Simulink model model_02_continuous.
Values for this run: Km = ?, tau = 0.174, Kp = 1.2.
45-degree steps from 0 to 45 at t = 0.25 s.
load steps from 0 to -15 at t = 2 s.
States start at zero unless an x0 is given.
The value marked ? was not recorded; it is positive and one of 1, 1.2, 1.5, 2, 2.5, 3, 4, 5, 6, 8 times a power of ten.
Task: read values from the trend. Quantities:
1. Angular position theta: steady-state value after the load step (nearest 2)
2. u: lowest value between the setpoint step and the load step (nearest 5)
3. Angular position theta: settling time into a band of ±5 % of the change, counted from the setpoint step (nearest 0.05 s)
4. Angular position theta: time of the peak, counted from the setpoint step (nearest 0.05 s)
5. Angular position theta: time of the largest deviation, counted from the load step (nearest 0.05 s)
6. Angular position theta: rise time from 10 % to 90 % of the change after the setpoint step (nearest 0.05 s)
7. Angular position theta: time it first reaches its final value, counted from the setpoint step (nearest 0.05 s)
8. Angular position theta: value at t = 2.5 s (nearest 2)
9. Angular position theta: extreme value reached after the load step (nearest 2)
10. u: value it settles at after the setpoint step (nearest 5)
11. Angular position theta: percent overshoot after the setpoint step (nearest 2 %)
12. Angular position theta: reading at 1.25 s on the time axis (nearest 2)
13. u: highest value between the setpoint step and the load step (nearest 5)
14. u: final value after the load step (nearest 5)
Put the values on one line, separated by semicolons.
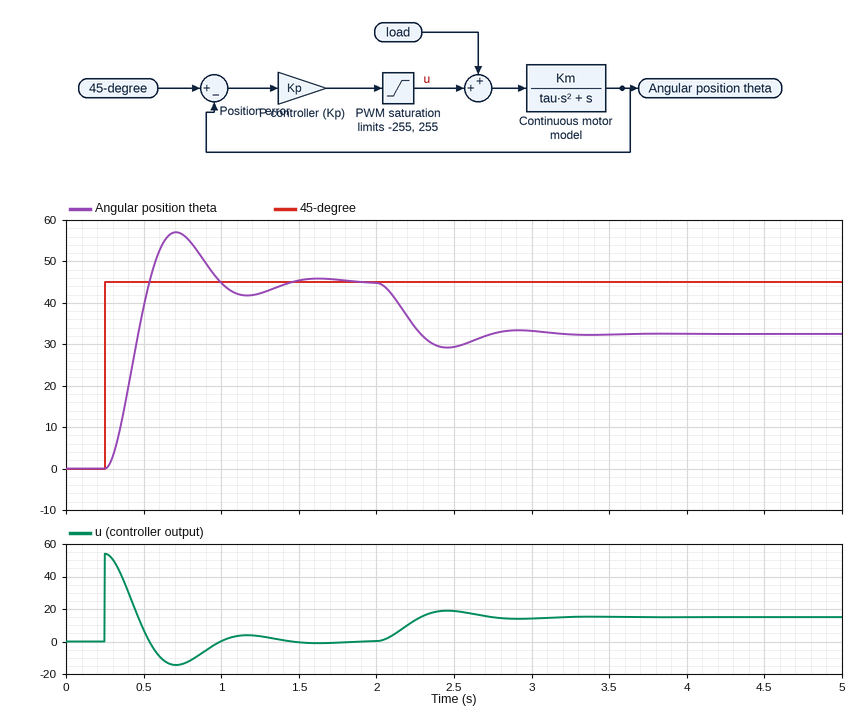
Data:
32; -15; 1.05 s; 0.45 s; 0.45 s; 0.20 s; 0.30 s; 30; 30; 0; 26 %; 42; 55; 15
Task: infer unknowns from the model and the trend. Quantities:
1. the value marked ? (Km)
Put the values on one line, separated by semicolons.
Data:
8
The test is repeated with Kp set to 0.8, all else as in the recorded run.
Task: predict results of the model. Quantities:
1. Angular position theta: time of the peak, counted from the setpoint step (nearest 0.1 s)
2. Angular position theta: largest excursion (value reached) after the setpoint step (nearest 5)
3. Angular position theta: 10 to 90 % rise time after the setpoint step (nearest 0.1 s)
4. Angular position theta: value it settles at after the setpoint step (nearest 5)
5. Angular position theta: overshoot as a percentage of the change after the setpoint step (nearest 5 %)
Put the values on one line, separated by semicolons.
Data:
0.6 s; 55; 0.3 s; 45; 20 %
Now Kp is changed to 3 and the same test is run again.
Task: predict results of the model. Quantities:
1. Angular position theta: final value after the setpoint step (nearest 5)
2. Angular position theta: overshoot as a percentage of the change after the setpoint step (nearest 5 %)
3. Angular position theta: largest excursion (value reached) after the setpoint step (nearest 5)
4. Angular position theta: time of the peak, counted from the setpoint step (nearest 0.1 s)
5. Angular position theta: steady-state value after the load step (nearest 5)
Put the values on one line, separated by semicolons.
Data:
45; 45 %; 65; 0.3 s; 40
